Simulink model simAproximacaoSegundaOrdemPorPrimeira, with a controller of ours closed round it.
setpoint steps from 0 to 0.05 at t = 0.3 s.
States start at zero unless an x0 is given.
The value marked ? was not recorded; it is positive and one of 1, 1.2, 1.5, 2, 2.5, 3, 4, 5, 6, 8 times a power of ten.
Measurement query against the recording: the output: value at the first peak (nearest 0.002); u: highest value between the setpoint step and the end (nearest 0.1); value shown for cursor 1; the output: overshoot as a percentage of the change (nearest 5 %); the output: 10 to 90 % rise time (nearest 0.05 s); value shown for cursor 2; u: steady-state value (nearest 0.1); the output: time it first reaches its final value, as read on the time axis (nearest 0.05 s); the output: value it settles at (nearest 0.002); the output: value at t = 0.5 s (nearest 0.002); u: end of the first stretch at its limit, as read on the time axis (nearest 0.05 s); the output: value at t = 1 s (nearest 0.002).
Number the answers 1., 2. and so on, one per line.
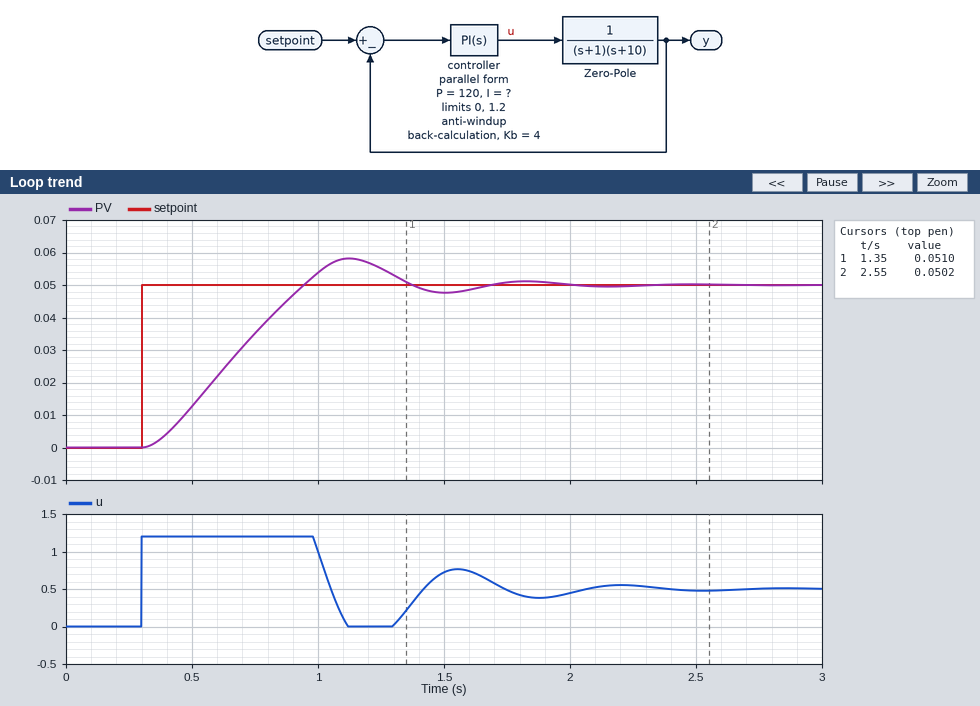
1. 0.058
2. 1.2
3. 0.0510
4. 15 %
5. 0.45 s
6. 0.0502
7. 0.5
8. 0.95 s
9. 0.050
10. 0.012
11. 1.00 s
12. 0.054
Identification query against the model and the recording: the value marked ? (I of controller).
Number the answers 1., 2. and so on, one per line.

1. 600
